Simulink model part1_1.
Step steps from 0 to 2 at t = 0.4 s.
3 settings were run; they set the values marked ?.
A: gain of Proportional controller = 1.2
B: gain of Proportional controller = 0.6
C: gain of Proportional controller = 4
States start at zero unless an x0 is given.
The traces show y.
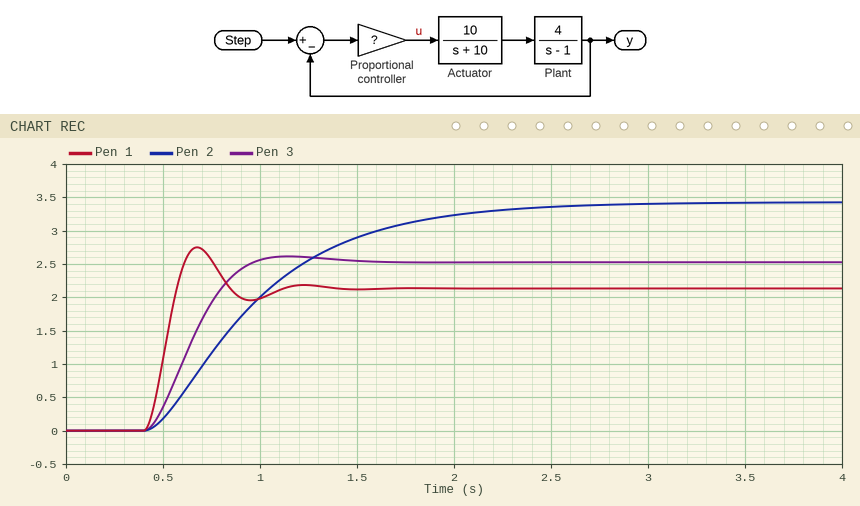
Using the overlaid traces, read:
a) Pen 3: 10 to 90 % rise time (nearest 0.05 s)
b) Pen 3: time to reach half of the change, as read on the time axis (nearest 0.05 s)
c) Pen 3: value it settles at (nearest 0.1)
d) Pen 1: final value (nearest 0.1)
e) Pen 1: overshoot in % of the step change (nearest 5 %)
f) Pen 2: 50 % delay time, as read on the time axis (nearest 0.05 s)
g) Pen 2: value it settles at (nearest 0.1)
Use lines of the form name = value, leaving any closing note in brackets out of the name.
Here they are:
Pen 3: 10 to 90 % rise time = 0.35 s
Pen 3: time to reach half of the change, as read on the time axis = 0.65 s
Pen 3: value it settles at = 2.5
Pen 1: final value = 2.1
Pen 1: overshoot in % of the step change = 30 %
Pen 2: 50 % delay time, as read on the time axis = 0.90 s
Pen 2: value it settles at = 3.4
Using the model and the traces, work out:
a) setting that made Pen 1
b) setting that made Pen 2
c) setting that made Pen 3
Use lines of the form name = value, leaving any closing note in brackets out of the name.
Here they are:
setting that made Pen 1 = C
setting that made Pen 2 = B
setting that made Pen 3 = A
